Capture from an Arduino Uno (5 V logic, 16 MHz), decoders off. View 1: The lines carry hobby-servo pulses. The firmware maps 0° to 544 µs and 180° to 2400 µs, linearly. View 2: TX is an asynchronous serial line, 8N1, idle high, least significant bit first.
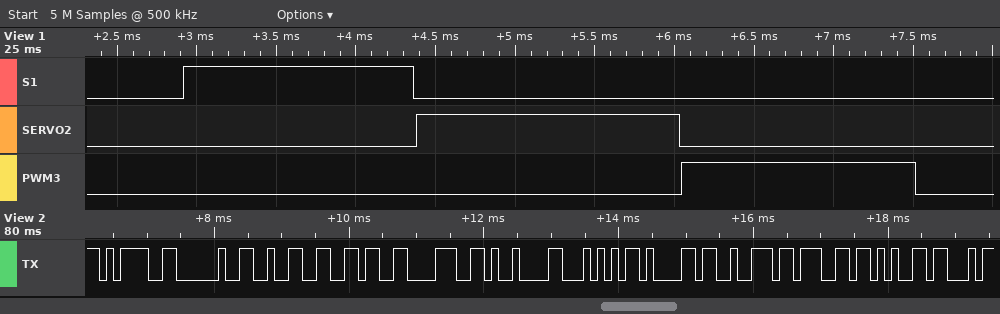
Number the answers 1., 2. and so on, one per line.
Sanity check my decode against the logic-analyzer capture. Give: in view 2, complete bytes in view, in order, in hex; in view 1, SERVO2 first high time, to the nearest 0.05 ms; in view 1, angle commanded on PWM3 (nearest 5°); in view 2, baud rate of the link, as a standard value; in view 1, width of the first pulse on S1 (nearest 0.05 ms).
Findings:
1. 0x3D 0x20 0x32 0x36 0x38 0x09 0x54 0x61 0x72 0x67 0x65
2. 1.65 ms
3. 90°
4. 9600 baud
5. 1.45 ms
